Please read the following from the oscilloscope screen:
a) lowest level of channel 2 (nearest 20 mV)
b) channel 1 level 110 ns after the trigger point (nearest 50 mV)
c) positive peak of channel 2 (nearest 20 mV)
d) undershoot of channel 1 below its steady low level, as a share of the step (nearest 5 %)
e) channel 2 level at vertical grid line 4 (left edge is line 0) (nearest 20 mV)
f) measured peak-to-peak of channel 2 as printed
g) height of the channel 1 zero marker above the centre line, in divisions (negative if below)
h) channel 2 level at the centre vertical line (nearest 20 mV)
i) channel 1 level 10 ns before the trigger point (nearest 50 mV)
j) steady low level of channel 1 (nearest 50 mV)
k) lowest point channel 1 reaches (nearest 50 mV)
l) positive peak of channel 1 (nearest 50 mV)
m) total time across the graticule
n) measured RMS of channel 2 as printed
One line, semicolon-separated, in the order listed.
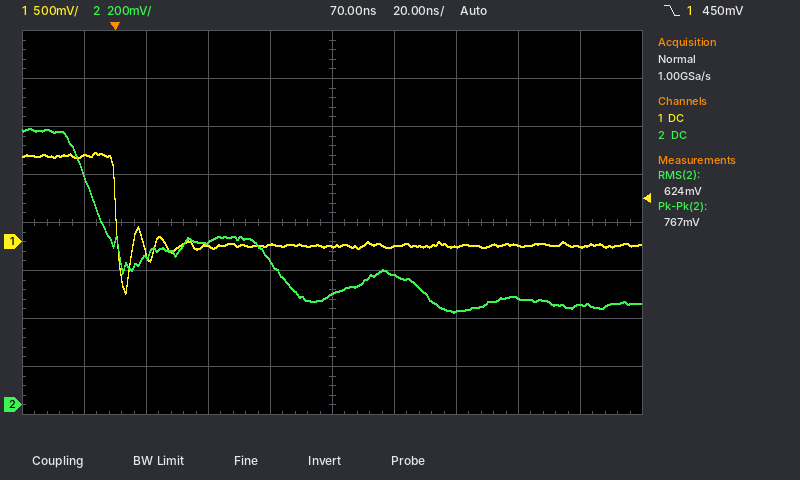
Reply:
380 mV; -50 mV; 1.16 V; 55 %; 600 mV; 767 mV; -0.4 div; 460 mV; 900 mV; -50 mV; -550 mV; 950 mV; 200 ns; 624 mV
